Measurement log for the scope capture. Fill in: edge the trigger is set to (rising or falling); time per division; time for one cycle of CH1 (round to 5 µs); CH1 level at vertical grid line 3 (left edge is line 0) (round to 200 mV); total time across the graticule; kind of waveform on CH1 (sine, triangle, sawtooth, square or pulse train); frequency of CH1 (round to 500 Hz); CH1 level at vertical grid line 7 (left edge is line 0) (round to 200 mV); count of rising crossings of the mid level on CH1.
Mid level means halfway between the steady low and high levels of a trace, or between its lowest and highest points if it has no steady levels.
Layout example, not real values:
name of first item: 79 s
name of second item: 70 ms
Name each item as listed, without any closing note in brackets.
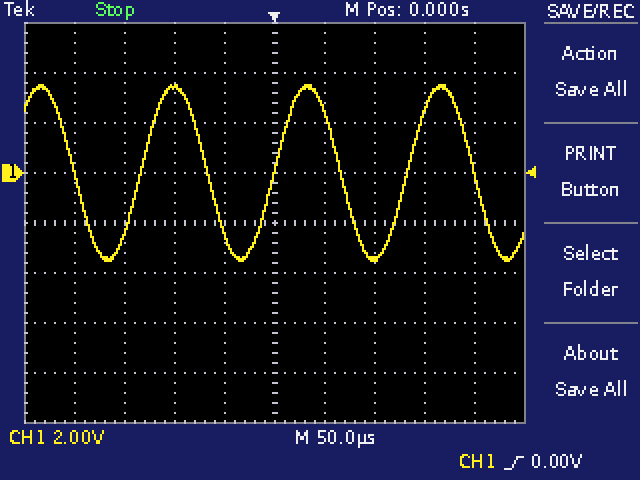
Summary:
edge the trigger is set to: rising
time per division: 50 µs
time for one cycle of CH1: 135 µs
CH1 level at vertical grid line 3 (left edge is line 0): 3.4 V
total time across the graticule: 500 µs
kind of waveform on CH1: sine
frequency of CH1: 7.5 kHz
CH1 level at vertical grid line 7 (left edge is line 0): -3.4 V
count of rising crossings of the mid level on CH1: 3
